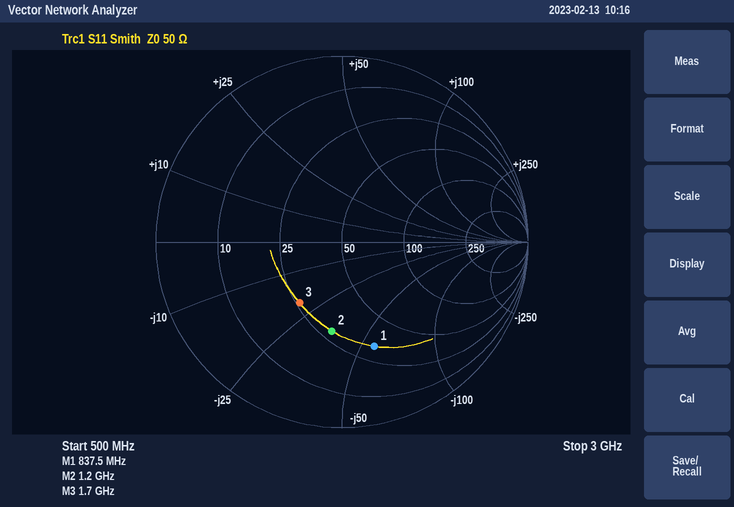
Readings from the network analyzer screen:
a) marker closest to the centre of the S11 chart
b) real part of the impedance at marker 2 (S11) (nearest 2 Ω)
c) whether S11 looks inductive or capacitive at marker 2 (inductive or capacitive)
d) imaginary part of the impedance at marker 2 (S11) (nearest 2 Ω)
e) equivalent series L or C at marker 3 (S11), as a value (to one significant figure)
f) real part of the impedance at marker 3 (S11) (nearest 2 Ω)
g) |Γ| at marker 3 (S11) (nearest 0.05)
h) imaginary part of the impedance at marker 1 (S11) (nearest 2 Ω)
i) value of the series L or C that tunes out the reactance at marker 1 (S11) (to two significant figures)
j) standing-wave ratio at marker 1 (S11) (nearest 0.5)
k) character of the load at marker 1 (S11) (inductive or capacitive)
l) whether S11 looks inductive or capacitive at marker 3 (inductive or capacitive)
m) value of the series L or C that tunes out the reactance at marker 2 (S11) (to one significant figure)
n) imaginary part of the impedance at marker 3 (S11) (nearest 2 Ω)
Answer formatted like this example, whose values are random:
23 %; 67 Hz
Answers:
marker 3; 28 Ω; capacitive; -36 Ω; 5 pF; 26 Ω; 0.40; -56 Ω; 11 nH; 4.0; capacitive; capacitive; 5 nH; -20 Ω
